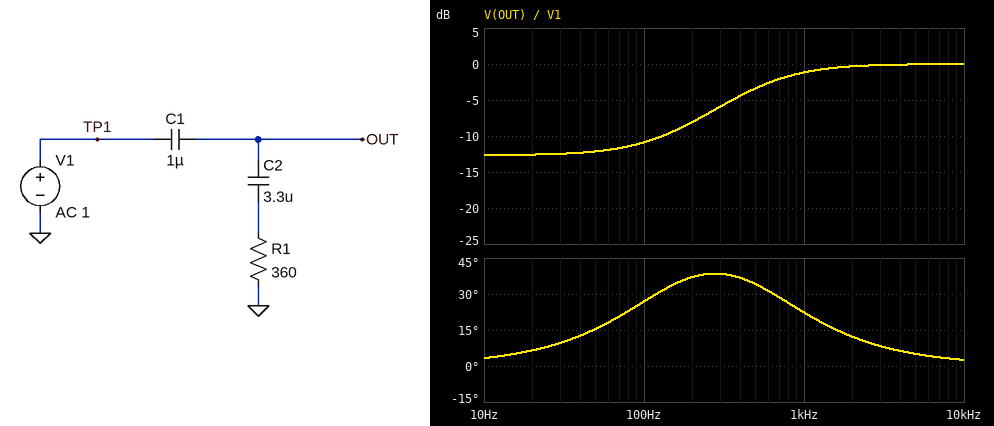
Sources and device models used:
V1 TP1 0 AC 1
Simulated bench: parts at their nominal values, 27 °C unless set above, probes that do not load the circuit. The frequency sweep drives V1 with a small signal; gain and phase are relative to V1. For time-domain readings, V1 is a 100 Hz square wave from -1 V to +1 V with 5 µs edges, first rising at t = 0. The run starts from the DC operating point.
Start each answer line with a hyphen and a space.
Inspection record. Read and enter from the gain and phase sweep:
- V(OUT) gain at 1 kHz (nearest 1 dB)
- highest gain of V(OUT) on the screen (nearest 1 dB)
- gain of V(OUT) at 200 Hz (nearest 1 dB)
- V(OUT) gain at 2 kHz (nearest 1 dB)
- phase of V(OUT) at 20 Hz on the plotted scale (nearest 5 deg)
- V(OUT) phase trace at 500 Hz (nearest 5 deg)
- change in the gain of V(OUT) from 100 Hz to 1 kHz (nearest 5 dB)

- -1 dB
- 0 dB
- -8 dB
- 0 dB
- 5 deg
- 35 deg
- 10 dB
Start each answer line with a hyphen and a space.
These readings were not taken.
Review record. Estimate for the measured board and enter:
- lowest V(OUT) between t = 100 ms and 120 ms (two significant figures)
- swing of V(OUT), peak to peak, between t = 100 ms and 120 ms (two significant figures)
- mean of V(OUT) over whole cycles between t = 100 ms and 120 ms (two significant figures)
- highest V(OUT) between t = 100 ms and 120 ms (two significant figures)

- -1.5 V
- 3.5 V
- 230 mV
- 2.0 V
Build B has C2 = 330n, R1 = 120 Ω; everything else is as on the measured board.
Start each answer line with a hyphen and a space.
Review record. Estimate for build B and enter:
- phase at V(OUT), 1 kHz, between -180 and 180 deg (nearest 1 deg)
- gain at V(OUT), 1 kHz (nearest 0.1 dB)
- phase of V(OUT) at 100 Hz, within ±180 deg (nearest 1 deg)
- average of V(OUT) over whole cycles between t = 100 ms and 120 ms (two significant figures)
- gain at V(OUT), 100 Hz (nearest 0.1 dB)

- 3 deg
- -2.4 dB
- 0 deg
- 750 mV
- -2.5 dB
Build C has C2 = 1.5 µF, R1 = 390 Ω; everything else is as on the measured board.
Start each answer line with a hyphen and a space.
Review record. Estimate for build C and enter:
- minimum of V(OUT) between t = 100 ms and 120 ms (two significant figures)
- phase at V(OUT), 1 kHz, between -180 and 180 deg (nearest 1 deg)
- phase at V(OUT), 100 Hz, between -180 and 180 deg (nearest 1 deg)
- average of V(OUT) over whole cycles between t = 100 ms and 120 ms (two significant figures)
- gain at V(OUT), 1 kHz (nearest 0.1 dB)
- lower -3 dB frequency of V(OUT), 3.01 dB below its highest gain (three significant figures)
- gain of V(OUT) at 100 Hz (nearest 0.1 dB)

- -1.2 V
- 19 deg
- 12 deg
- 400 mV
- -1.3 dB
- 561 Hz
- -7.5 dB
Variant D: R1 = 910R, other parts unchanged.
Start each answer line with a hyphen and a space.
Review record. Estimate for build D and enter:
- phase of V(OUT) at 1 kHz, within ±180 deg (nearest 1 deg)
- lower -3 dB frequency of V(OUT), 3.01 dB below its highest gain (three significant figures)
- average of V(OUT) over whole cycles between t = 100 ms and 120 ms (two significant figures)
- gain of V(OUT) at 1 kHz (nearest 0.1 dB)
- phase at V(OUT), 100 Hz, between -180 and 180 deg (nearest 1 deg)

- 10 deg
- 215 Hz
- 230 mV
- -0.2 dB
- 38 deg
